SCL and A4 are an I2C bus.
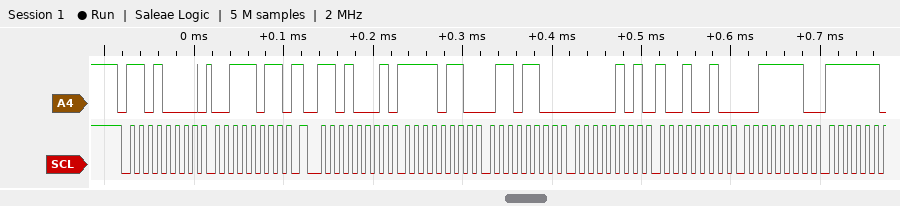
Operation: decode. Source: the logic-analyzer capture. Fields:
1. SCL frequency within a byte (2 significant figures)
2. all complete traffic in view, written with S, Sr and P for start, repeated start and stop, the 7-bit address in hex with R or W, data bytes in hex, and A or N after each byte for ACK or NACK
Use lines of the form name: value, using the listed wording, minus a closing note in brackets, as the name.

SCL frequency within a byte: 100 kHz
all complete traffic in view, written with S, Sr and P for start, repeated start and stop, the 7-bit address in hex with R or W, data bytes in hex, and A or N after each byte for ACK or NACK: S 68W A 3B A Sr 68R A F6 A 6C A 05 A 92 A 3E A
